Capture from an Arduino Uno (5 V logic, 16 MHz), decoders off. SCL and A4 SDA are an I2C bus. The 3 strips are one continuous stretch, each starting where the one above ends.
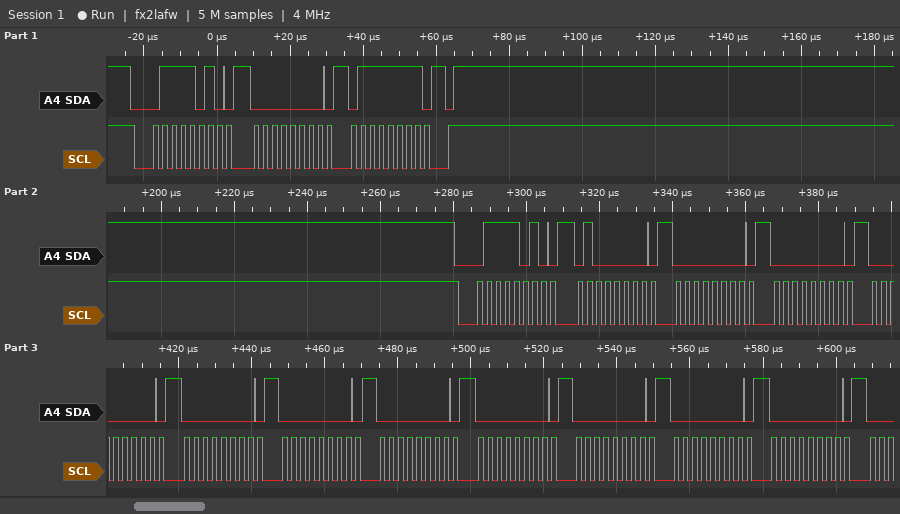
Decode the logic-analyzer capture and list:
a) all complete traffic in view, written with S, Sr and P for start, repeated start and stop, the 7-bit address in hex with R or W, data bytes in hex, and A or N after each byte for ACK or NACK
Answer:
S 3DW A 00 A 7F A P S 3DW A 40 A 00 A 00 A 00 A 00 A 00 A 00 A 00 A 00 A 00 A 00 A
